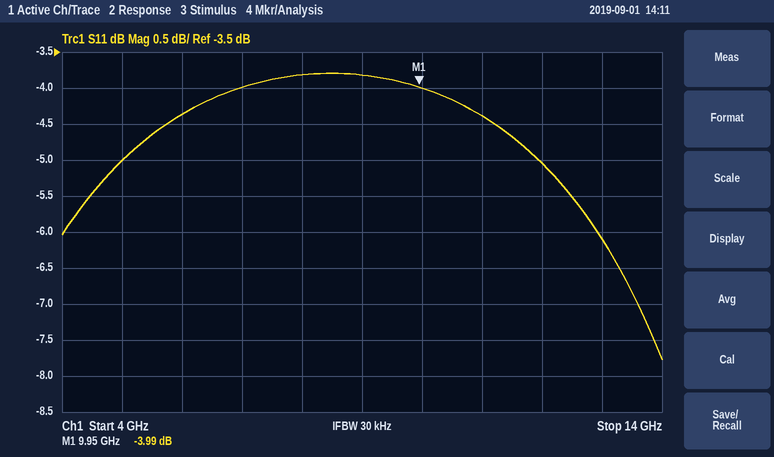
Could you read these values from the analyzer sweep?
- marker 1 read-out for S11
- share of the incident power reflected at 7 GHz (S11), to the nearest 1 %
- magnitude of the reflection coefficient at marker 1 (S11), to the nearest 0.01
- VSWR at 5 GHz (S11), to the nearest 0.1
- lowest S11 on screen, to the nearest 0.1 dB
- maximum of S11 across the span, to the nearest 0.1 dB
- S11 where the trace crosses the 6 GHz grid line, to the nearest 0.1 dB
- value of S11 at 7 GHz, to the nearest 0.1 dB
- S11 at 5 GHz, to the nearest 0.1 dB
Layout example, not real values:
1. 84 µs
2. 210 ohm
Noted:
1. -3.99 dB
2. 40 %
3. 0.63
4. 3.6
5. -7.8 dB
6. -3.8 dB
7. -4.4 dB
8. -4.0 dB
9. -5.0 dB
